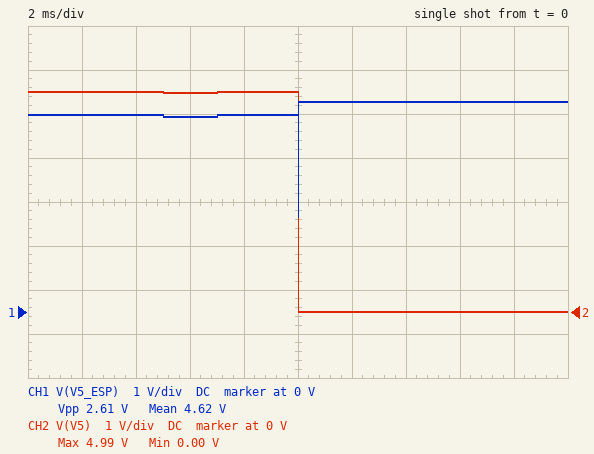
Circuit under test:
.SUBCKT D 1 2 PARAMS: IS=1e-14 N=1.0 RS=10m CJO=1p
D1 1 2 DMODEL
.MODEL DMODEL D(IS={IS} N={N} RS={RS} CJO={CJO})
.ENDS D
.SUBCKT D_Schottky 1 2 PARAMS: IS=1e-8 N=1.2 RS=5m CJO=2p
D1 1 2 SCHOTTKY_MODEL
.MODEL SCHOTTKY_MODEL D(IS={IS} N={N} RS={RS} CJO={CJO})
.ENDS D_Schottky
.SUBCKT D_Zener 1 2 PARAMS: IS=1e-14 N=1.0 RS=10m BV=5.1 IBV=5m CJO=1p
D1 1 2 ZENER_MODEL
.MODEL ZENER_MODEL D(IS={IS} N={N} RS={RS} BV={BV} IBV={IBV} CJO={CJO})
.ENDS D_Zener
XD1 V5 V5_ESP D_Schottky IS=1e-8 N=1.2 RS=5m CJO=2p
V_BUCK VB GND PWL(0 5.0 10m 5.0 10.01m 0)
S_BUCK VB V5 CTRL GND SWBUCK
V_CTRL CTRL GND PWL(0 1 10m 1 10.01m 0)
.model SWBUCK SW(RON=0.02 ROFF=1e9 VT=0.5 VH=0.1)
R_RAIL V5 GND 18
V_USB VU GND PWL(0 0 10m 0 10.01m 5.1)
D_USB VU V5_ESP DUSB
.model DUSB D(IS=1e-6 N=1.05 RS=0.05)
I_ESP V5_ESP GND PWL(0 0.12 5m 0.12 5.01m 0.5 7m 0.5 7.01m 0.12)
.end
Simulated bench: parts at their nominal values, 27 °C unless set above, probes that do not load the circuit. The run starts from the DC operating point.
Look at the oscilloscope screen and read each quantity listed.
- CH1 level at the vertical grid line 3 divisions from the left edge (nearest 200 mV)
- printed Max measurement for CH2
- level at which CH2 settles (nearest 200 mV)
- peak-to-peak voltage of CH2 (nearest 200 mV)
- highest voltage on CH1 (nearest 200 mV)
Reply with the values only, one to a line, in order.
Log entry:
4.4 V
4.99 V
0 V
5.0 V
4.8 V
